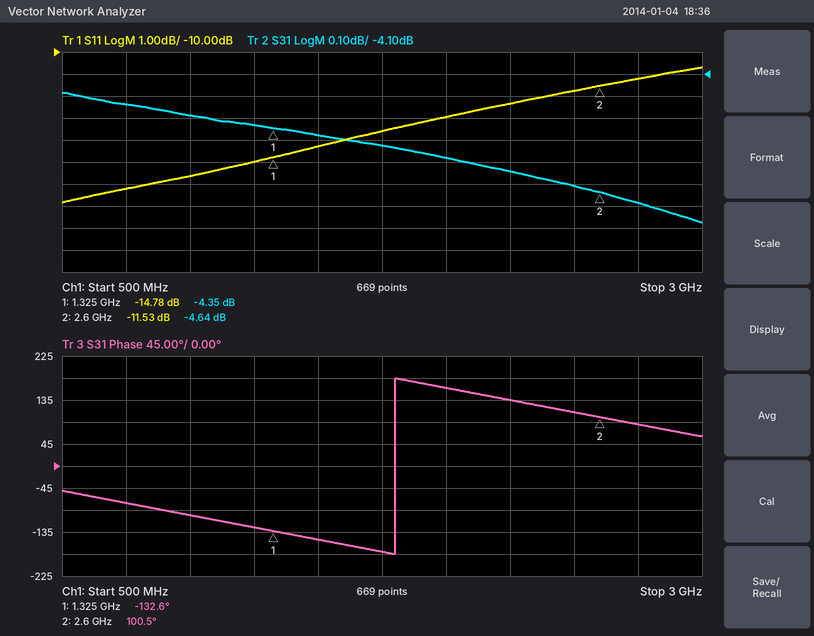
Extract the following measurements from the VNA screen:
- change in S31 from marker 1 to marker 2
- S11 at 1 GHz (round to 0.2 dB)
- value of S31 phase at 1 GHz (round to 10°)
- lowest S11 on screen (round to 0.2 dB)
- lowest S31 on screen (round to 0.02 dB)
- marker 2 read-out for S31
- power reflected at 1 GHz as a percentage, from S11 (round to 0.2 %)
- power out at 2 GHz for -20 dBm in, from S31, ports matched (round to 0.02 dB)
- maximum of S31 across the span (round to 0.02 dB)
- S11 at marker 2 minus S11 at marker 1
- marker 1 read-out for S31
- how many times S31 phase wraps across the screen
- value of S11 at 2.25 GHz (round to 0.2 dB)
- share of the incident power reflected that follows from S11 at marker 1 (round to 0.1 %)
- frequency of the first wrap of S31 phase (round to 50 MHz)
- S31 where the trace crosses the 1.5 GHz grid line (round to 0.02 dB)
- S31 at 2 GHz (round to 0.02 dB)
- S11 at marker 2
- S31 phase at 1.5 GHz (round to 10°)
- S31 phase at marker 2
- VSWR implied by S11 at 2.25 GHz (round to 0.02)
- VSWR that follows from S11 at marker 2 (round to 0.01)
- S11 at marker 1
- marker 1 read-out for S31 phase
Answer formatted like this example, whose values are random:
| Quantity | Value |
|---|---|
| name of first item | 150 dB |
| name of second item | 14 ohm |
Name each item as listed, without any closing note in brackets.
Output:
| Quantity | Value |
|---|---|
| change in S31 from marker 1 to marker 2 | -0.29 dB |
| S11 at 1 GHz | -15.6 dB |
| value of S31 phase at 1 GHz | -100° |
| lowest S11 on screen | -16.8 dB |
| lowest S31 on screen | -4.78 dB |
| marker 2 read-out for S31 | -4.64 dB |
| power reflected at 1 GHz as a percentage, from S11 | 2.8 % |
| power out at 2 GHz for -20 dBm in, from S31, ports matched | -24.48 dBm |
| maximum of S31 across the span | -4.18 dB |
| S11 at marker 2 minus S11 at marker 1 | 3.25 dB |
| marker 1 read-out for S31 | -4.35 dB |
| how many times S31 phase wraps across the screen | 1 |
| value of S11 at 2.25 GHz | -12.4 dB |
| share of the incident power reflected that follows from S11 at marker 1 | 3.3 % |
| frequency of the first wrap of S31 phase | 1.80 GHz |
| S31 where the trace crosses the 1.5 GHz grid line | -4.38 dB |
| S31 at 2 GHz | -4.48 dB |
| S11 at marker 2 | -11.53 dB |
| S31 phase at 1.5 GHz | -150° |
| S31 phase at marker 2 | 100.5° |
| VSWR implied by S11 at 2.25 GHz | 1.64 |
| VSWR that follows from S11 at marker 2 | 1.72 |
| S11 at marker 1 | -14.78 dB |
| marker 1 read-out for S31 phase | -132.6° |
